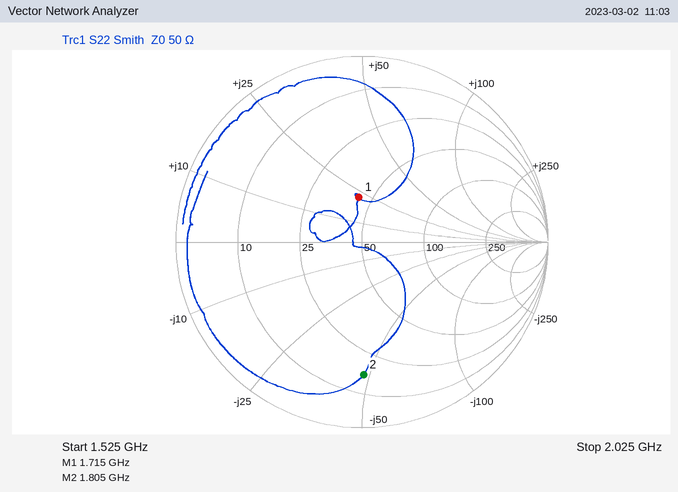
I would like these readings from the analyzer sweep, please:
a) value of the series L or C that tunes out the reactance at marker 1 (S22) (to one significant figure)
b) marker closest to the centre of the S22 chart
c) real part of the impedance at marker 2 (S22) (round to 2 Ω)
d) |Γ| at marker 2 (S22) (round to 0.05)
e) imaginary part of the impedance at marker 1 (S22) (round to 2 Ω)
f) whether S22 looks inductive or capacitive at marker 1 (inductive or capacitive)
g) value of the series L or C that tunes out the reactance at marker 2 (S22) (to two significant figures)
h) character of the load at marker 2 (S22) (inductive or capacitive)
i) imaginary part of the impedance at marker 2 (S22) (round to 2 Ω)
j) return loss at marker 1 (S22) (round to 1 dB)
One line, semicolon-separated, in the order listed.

4 pF; marker 1; 16 Ω; 0.70; +22 Ω; inductive; 4.2 nH; capacitive; -48 Ω; 12 dB
